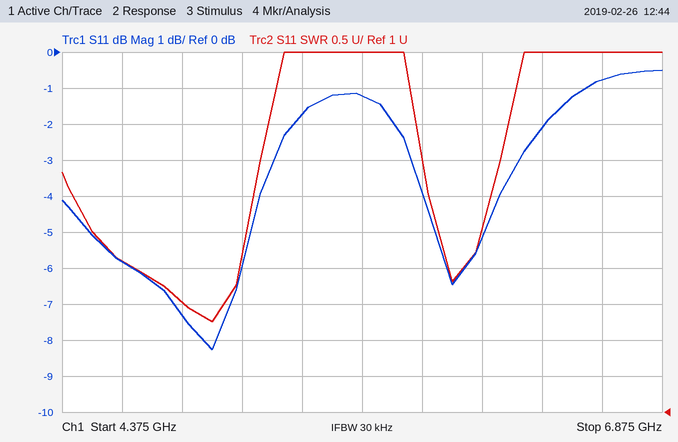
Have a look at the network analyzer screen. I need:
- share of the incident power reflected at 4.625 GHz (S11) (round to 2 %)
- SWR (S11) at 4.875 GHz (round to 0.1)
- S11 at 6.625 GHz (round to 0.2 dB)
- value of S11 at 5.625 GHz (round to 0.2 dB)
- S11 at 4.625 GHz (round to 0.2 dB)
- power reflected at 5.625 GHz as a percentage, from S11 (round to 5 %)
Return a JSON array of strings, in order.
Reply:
["26 %", "2.5", "-0.8 dB", "-1.2 dB", "-5.8 dB", "75 %"]
